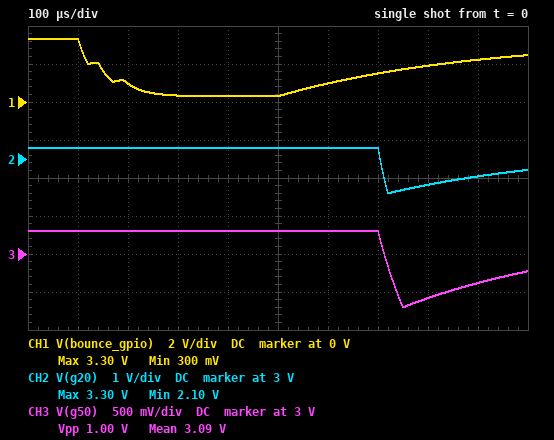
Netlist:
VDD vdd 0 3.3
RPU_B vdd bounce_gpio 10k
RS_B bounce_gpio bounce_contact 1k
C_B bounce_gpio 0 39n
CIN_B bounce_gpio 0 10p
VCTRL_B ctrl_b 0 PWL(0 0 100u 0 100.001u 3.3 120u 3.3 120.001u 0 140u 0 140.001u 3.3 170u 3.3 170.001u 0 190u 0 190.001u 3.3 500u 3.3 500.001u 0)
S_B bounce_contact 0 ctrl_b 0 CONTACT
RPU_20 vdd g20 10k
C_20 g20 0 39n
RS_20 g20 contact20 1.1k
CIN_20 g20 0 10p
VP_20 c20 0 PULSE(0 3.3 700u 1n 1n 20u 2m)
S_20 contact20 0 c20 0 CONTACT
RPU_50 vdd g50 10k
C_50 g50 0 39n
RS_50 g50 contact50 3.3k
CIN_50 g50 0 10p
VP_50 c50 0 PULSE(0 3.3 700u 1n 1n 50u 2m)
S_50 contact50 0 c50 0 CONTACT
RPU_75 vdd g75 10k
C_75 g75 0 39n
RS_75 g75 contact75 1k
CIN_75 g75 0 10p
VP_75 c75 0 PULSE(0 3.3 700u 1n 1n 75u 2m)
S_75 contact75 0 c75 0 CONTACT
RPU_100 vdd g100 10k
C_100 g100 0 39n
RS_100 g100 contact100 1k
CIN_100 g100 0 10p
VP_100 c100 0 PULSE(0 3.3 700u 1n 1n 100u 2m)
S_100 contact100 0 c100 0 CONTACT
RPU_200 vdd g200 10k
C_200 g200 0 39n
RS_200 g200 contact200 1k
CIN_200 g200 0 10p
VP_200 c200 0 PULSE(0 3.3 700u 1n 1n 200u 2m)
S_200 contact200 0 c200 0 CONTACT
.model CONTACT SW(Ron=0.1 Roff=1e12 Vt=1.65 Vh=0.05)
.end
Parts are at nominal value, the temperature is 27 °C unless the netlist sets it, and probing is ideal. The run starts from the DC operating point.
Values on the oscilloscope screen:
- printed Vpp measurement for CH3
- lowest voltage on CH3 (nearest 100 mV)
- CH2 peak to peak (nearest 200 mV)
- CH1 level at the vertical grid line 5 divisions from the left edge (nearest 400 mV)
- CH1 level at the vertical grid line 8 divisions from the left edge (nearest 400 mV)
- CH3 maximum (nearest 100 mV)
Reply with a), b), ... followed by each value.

a) 1.00 V
b) 2.3 V
c) 1.2 V
d) 400 mV
e) 2.0 V
f) 3.3 V
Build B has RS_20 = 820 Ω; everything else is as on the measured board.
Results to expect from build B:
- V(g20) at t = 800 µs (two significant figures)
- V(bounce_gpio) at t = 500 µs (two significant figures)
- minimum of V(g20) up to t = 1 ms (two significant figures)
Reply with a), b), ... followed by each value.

a) 2.1 V
b) 300 mV
c) 1.8 V
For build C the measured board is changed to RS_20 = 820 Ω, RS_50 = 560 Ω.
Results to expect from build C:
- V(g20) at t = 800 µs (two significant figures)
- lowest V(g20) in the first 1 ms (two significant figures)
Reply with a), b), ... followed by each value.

a) 2.1 V
b) 1.8 V
